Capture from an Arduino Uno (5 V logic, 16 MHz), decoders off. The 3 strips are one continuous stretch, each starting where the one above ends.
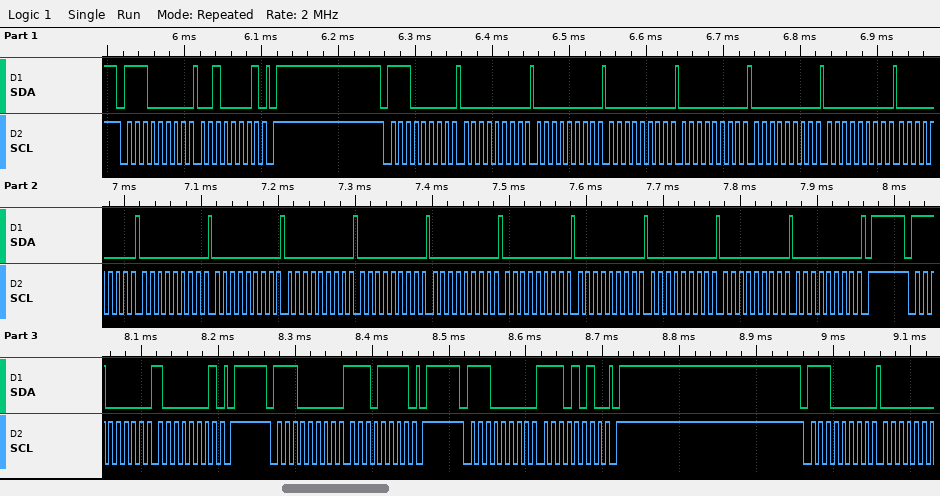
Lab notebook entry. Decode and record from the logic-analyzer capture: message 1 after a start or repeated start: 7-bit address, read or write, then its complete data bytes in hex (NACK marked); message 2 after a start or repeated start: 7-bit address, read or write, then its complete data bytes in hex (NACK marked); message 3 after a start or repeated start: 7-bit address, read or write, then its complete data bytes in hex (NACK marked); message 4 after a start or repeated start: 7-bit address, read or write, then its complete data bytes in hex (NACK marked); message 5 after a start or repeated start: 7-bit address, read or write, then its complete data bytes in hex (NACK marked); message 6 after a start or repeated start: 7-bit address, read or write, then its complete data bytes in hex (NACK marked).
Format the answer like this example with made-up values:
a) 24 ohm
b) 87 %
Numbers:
a) 0x70 write: 21
b) 0x70 write: 00 00 00 00 00 00 00 00 00 00 00 00 00 00 00 00 00
c) 0x70 write: 81
d) 0x70 write: EF
e) 0x70 write: EA
f) 0x70 write
